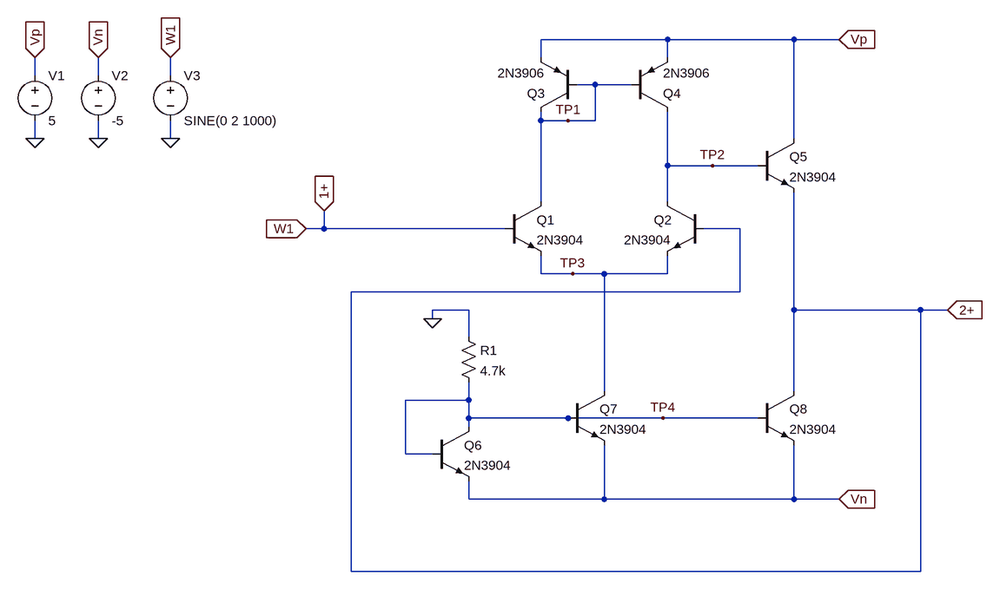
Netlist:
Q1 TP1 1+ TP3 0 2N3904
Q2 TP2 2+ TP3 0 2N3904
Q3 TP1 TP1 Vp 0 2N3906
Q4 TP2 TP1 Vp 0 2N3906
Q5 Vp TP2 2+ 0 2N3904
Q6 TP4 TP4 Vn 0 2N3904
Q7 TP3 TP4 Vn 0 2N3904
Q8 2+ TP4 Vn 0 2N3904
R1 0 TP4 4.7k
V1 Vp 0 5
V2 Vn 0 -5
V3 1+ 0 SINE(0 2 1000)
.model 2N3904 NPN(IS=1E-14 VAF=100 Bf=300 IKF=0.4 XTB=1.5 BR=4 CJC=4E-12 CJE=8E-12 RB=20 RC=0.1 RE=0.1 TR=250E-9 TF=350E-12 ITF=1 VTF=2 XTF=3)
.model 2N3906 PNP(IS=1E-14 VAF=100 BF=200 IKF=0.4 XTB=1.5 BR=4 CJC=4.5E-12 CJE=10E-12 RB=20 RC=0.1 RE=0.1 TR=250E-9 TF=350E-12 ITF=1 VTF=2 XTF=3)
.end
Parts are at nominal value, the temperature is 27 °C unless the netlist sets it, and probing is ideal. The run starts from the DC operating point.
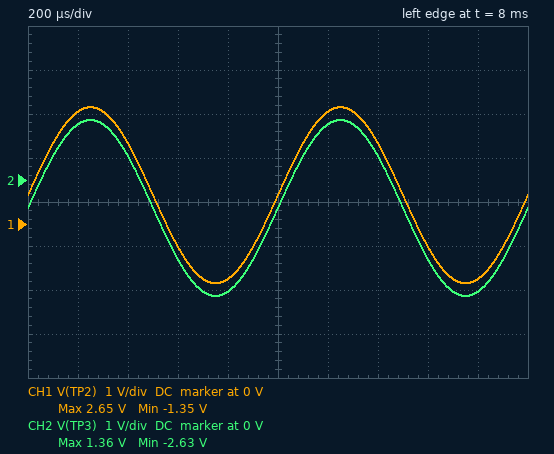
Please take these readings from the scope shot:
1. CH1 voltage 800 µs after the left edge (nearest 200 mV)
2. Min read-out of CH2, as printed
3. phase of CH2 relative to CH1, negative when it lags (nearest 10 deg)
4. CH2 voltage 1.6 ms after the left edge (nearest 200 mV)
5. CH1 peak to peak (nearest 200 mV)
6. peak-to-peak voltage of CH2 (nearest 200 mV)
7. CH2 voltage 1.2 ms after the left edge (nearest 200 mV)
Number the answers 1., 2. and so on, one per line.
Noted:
1. -1.2 V
2. -2.63 V
3. 0 deg
4. -1.8 V
5. 4.0 V
6. 4.0 V
7. 1.2 V
